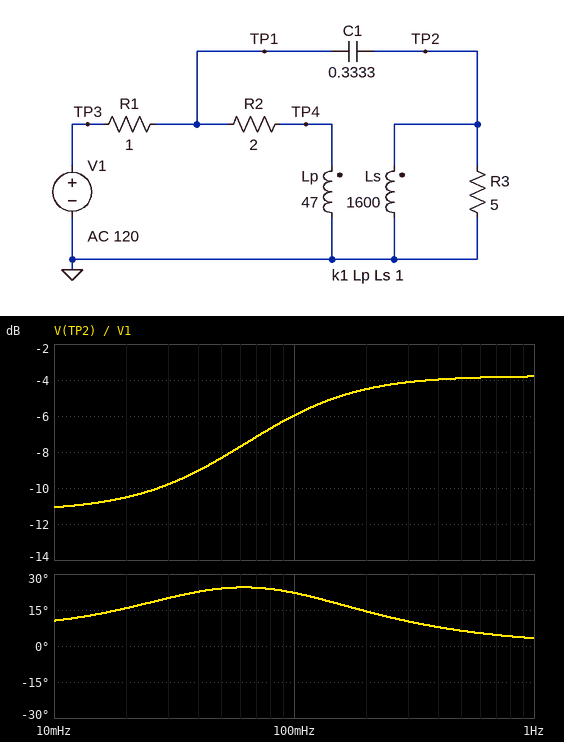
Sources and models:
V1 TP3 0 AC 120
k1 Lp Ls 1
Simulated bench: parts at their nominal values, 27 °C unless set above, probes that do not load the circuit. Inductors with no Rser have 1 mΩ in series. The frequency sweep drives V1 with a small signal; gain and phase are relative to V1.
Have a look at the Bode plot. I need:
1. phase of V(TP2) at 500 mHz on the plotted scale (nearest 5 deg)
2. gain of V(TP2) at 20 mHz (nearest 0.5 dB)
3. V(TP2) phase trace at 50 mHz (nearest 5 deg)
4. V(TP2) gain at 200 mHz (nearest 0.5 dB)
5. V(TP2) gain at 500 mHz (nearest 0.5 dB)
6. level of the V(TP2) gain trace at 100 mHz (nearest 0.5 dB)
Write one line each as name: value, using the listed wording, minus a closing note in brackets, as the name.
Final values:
phase of V(TP2) at 500 mHz on the plotted scale: 5 deg
gain of V(TP2) at 20 mHz: -10.5 dB
V(TP2) phase trace at 50 mHz: 25 deg
V(TP2) gain at 200 mHz: -4.5 dB
V(TP2) gain at 500 mHz: -4.0 dB
level of the V(TP2) gain trace at 100 mHz: -6.0 dB
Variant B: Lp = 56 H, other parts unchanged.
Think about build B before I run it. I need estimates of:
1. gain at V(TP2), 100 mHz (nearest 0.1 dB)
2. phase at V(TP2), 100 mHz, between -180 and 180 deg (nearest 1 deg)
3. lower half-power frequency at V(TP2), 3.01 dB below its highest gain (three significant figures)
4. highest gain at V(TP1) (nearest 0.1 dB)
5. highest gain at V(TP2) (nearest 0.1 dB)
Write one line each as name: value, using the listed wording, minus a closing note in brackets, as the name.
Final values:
gain at V(TP2), 100 mHz: -5.9 dB
phase at V(TP2), 100 mHz, between -180 and 180 deg: 21 deg
lower half-power frequency at V(TP2), 3.01 dB below its highest gain: 75.8 mHz
highest gain at V(TP1): -3.3 dB
highest gain at V(TP2): -3.7 dB
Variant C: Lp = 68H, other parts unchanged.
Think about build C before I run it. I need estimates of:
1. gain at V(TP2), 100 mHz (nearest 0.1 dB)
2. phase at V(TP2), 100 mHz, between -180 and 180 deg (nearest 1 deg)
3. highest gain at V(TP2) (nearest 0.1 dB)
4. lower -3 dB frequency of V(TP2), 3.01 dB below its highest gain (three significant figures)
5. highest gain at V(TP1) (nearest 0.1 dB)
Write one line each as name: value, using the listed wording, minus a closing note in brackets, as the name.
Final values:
gain at V(TP2), 100 mHz: -5.7 dB
phase at V(TP2), 100 mHz, between -180 and 180 deg: 19 deg
highest gain at V(TP2): -3.6 dB
lower -3 dB frequency of V(TP2), 3.01 dB below its highest gain: 73.0 mHz
highest gain at V(TP1): -3.2 dB
